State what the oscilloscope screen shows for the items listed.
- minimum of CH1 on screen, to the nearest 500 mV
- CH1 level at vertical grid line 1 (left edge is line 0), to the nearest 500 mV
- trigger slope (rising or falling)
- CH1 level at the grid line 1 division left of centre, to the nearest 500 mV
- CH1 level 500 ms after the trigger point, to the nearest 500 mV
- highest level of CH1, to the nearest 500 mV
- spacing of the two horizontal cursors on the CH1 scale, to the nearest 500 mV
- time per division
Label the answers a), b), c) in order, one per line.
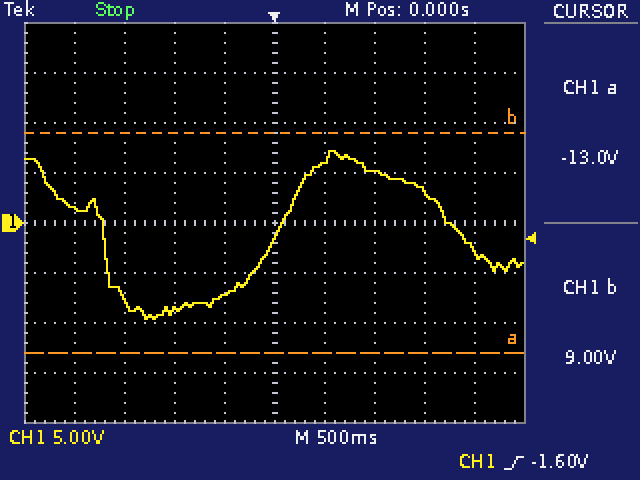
a) -9.5 V
b) 1.5 V
c) rising
d) -7.0 V
e) 6.0 V
f) 7.0 V
g) 22.0 V
h) 500 ms
